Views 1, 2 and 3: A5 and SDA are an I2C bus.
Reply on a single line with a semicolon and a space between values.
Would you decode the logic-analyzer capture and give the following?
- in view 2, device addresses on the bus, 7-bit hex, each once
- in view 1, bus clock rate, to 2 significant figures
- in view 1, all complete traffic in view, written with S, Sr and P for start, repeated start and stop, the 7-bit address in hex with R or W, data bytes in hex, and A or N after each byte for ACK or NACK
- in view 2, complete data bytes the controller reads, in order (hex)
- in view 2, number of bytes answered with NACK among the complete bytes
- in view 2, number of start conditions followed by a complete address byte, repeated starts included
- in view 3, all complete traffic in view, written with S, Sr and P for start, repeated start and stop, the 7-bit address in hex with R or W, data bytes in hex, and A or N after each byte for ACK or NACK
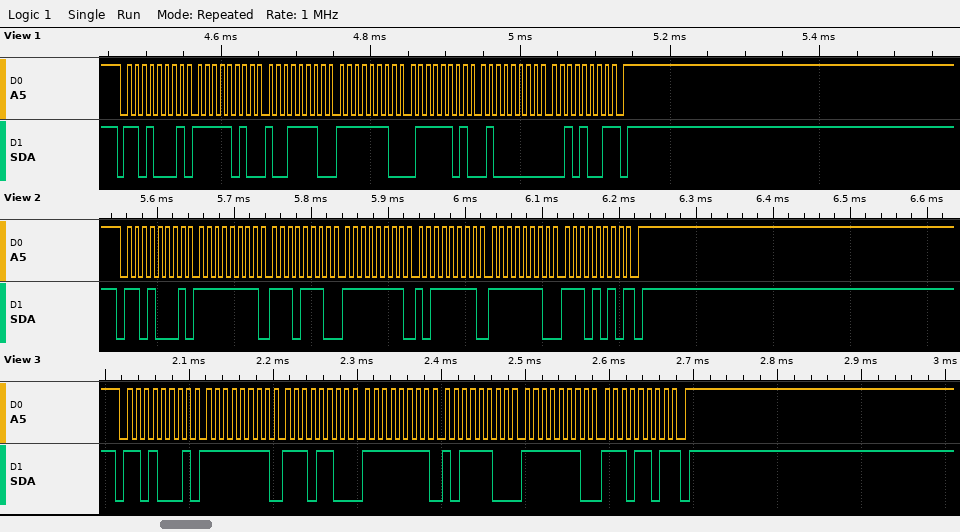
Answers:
0x68; 100 kHz; S 68R A FA A 9E A FE A 7D A 40 A 29 N P; FF EE FF BF FE EA; 1; 1; S 68R A FF A EC A FF A BC A FE A ED N P
